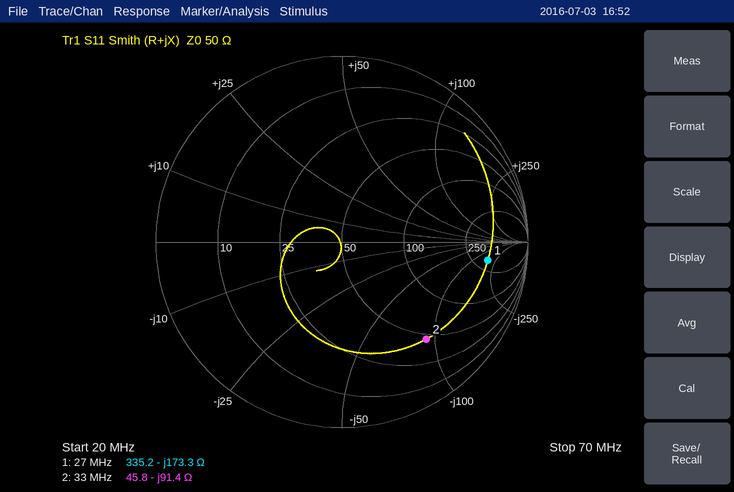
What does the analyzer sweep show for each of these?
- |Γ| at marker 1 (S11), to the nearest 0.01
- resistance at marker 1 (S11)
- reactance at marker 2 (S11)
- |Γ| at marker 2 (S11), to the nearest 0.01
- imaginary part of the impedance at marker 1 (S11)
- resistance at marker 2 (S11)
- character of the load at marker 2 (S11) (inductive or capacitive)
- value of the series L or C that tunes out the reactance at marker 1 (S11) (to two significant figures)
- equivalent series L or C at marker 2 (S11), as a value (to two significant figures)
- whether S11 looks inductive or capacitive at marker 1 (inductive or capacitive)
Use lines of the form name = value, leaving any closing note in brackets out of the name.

|Γ| at marker 1 (S11), to the nearest 0.01 = 0.79
resistance at marker 1 = 335.2 Ω
reactance at marker 2 = -91.4 Ω
|Γ| at marker 2 (S11), to the nearest 0.01 = 0.69
imaginary part of the impedance at marker 1 = -173.3 Ω
resistance at marker 2 = 45.8 Ω
character of the load at marker 2 (S11) = capacitive
value of the series L or C that tunes out the reactance at marker 1 (S11) = 1.0 µH
equivalent series L or C at marker 2 (S11), as a value = 53 pF
whether S11 looks inductive or capacitive at marker 1 = capacitive
